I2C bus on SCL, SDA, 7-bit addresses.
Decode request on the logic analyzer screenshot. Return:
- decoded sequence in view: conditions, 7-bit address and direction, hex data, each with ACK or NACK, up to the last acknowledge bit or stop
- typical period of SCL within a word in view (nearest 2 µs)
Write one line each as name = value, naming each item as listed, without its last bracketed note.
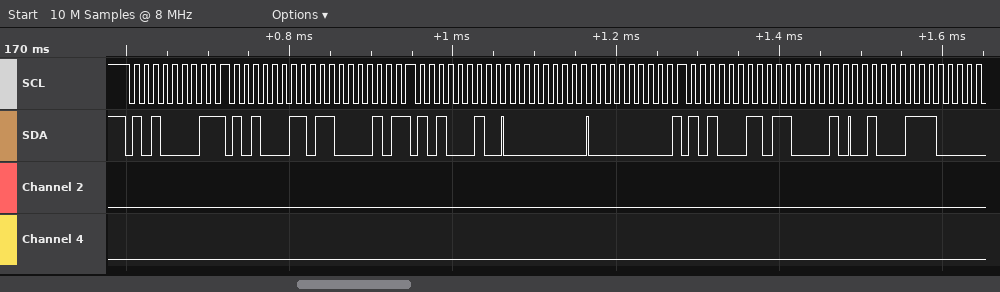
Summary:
decoded sequence in view: conditions, 7-bit address and direction, hex data, each with ACK or NACK, up to the last acknowledge bit or stop = start, address 50 read NACK, repeated start, address 51 read ACK, C2 NACK, repeated start, address 51 write ACK, 00 ACK, 00 ACK, repeated start, address 51 read ACK, C2 ACK, 47 ACK
typical period of SCL within a word in view = 12 µs
